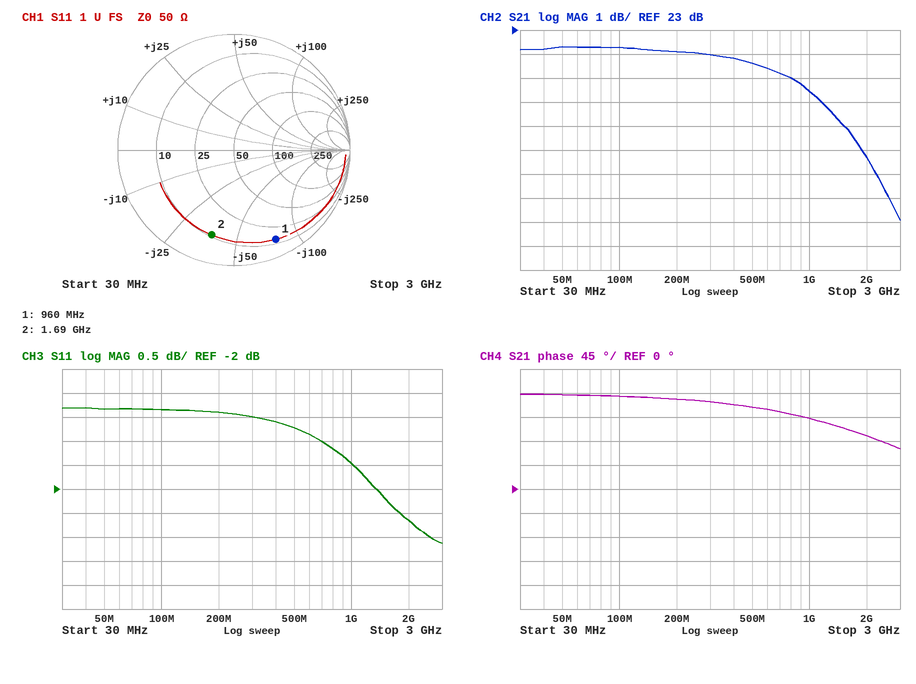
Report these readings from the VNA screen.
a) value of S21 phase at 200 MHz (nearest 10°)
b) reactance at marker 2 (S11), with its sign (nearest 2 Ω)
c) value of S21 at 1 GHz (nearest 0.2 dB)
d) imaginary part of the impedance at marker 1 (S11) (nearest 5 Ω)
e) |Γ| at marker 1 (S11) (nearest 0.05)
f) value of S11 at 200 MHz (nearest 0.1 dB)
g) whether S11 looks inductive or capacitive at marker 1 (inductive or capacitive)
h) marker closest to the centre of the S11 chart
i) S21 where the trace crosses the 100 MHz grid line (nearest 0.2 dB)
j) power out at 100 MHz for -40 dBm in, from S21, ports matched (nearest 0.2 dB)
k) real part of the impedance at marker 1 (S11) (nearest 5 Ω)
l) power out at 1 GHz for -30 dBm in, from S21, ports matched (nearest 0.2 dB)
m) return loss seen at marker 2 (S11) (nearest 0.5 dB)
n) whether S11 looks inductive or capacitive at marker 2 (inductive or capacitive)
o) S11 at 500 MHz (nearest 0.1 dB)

170°
-38 Ω
20.4 dB
-75 Ω
0.85
-0.4 dB
capacitive
marker 2
22.2 dB
-17.8 dBm
15 Ω
-9.6 dBm
2.5 dB
capacitive
-0.7 dB
